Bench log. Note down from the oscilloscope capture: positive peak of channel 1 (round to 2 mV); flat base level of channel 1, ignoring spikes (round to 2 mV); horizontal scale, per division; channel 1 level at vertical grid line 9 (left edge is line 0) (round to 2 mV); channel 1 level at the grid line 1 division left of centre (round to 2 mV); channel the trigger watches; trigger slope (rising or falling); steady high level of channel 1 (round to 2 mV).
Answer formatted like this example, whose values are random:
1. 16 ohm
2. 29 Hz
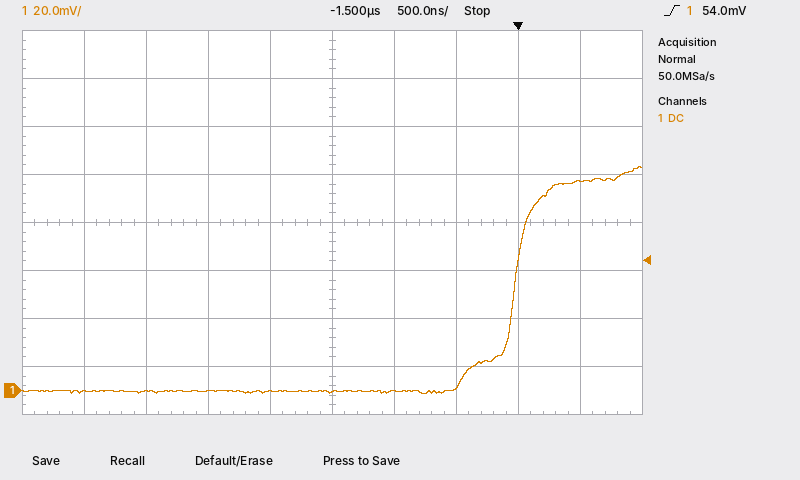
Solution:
1. 94 mV
2. 0 mV
3. 500 ns
4. 88 mV
5. 0 mV
6. channel 1
7. rising
8. 88 mV
